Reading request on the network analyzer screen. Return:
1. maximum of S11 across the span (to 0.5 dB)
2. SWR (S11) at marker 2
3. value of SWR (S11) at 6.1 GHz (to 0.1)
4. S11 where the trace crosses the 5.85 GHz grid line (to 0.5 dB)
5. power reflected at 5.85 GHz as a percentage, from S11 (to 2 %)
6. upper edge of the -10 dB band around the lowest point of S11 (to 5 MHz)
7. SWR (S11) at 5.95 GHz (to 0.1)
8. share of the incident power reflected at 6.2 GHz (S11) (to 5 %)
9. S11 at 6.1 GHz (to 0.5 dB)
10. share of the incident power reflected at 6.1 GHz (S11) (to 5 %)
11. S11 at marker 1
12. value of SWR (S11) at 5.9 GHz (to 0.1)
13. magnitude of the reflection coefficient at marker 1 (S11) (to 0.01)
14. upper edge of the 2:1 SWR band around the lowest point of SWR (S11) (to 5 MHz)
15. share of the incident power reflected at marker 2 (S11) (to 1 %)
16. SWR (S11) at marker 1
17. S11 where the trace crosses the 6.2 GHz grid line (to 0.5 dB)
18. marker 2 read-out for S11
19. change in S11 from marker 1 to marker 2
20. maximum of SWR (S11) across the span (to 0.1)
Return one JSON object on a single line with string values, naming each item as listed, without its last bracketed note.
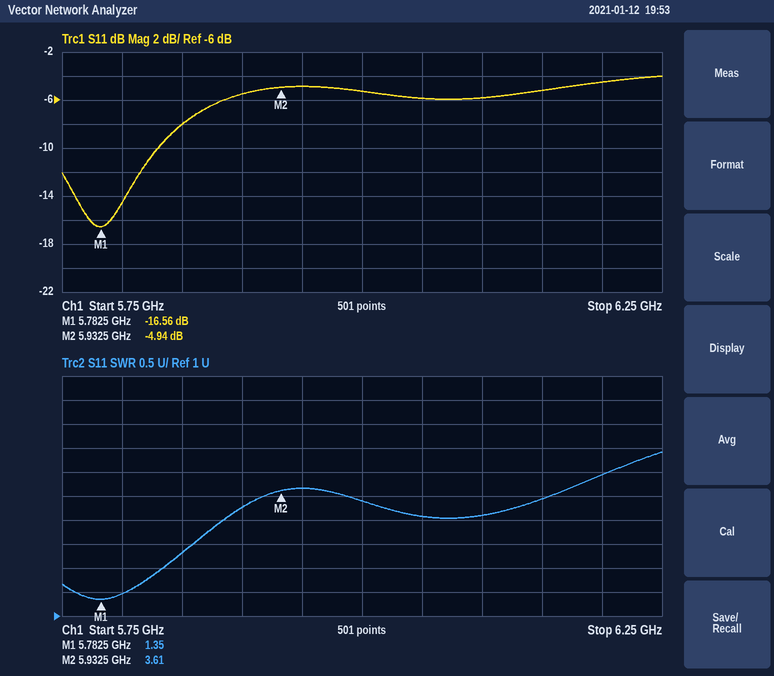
{"maximum of S11 across the span": "-4.0 dB", "SWR (S11) at marker 2": "3.61", "value of SWR (S11) at 6.1 GHz": "3.1", "S11 where the trace crosses the 5.85 GHz grid line": "-8.0 dB", "power reflected at 5.85 GHz as a percentage, from S11": "16 %", "upper edge of the -10 dB band around the lowest point of S11": "5.830 GHz", "SWR (S11) at 5.95 GHz": "3.7", "share of the incident power reflected at 6.2 GHz (S11)": "35 %", "S11 at 6.1 GHz": "-6.0 dB", "share of the incident power reflected at 6.1 GHz (S11)": "25 %", "S11 at marker 1": "-16.56 dB", "value of SWR (S11) at 5.9 GHz": "3.3", "magnitude of the reflection coefficient at marker 1 (S11)": "0.15", "upper edge of the 2:1 SWR band around the lowest point of SWR (S11)": "5.835 GHz", "share of the incident power reflected at marker 2 (S11)": "32 %", "SWR (S11) at marker 1": "1.35", "S11 where the trace crosses the 6.2 GHz grid line": "-4.5 dB", "marker 2 read-out for S11": "-4.94 dB", "change in S11 from marker 1 to marker 2": "11.62 dB", "maximum of SWR (S11) across the span": "4.4"}
